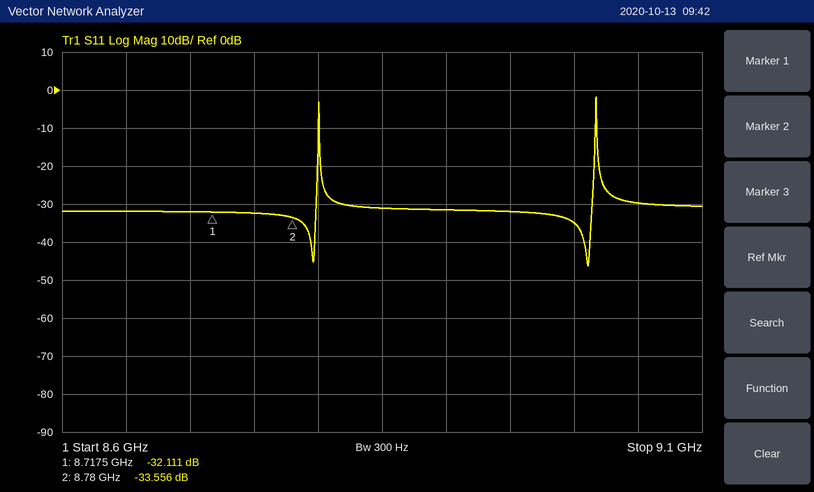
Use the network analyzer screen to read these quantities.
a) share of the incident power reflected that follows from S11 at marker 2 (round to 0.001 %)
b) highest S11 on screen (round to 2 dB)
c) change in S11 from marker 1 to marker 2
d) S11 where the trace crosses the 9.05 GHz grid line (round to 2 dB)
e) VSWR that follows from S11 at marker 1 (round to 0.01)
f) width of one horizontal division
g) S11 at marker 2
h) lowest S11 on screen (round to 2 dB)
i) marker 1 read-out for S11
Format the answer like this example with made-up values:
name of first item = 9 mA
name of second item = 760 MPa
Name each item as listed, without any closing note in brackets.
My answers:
share of the incident power reflected that follows from S11 at marker 2 = 0.044 %
highest S11 on screen = -2 dB
change in S11 from marker 1 to marker 2 = -1.445 dB
S11 where the trace crosses the 9.05 GHz grid line = -30 dB
VSWR that follows from S11 at marker 1 = 1.05
width of one horizontal division = 50 MHz
S11 at marker 2 = -33.556 dB
lowest S11 on screen = -46 dB
marker 1 read-out for S11 = -32.111 dB
